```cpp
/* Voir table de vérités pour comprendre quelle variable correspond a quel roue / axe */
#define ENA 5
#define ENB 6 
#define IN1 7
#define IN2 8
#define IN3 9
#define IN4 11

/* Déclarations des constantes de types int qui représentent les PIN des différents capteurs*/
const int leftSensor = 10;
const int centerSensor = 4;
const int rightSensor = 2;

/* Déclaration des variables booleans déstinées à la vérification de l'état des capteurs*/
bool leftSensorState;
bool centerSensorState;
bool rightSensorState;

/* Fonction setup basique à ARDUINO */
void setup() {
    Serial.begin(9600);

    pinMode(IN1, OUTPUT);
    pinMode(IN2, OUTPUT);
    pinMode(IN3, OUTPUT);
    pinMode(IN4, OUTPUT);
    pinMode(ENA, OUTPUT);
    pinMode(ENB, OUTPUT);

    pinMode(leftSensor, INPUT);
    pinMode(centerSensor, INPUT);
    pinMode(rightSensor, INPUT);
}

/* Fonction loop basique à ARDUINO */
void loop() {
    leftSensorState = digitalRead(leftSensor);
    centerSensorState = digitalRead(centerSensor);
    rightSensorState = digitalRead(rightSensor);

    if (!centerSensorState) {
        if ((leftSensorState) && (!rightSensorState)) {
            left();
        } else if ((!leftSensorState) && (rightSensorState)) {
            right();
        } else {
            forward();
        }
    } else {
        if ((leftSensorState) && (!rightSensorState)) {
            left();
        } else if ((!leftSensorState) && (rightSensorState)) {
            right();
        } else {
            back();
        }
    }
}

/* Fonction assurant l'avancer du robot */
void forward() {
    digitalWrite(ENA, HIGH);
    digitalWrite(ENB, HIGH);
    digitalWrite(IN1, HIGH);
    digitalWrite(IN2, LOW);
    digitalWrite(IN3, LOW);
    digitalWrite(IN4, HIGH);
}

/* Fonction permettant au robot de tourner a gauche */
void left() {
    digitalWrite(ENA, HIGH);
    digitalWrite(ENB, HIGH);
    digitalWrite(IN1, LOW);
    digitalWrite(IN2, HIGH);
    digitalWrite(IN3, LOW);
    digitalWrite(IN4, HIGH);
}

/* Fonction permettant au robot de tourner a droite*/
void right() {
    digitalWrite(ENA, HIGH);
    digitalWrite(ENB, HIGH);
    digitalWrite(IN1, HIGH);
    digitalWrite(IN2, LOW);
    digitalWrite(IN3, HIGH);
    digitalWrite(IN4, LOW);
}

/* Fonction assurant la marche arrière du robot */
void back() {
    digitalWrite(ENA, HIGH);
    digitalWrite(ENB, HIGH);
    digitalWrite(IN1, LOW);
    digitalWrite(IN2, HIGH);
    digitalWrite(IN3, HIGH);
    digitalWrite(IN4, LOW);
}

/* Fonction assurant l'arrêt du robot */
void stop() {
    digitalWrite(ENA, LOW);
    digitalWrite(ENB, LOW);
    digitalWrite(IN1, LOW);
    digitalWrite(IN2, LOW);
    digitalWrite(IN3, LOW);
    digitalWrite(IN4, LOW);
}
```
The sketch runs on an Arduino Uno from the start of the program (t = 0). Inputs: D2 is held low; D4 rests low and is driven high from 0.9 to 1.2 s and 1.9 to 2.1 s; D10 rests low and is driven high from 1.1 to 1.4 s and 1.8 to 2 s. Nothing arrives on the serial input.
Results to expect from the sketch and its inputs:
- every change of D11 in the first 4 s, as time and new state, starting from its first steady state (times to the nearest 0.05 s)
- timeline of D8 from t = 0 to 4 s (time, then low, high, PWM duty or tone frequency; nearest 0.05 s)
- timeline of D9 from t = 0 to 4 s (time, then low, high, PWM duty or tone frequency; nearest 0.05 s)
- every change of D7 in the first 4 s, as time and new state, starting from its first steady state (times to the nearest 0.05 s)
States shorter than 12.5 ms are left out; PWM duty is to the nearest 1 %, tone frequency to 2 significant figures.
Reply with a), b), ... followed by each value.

a) 0 s high; 0.9 s low; 1.1 s high; 2 s low; 2.1 s high
b) 0 s low; 0.9 s high; 1.4 s low; 1.8 s high; 2.1 s low
c) 0 s low; 0.9 s high; 1.1 s low; 2 s high; 2.1 s low
d) 0 s high; 0.9 s low; 1.4 s high; 1.8 s low; 2.1 s high
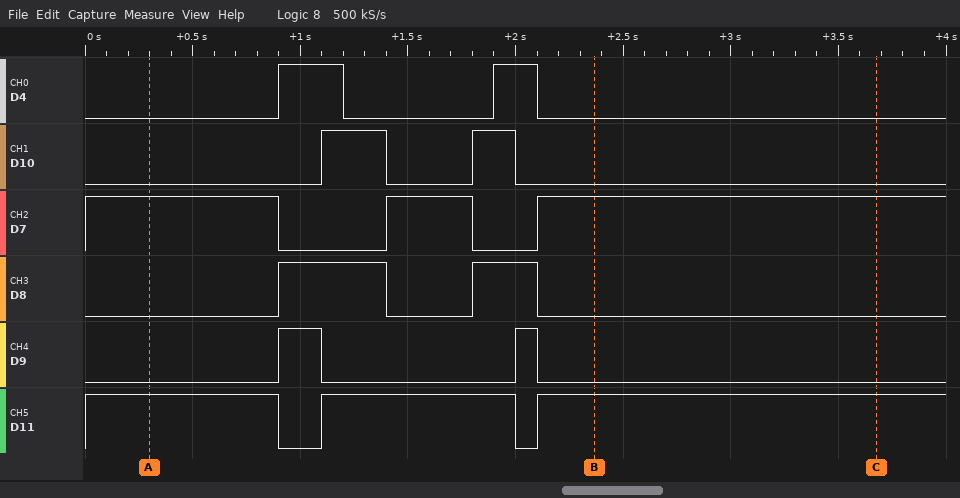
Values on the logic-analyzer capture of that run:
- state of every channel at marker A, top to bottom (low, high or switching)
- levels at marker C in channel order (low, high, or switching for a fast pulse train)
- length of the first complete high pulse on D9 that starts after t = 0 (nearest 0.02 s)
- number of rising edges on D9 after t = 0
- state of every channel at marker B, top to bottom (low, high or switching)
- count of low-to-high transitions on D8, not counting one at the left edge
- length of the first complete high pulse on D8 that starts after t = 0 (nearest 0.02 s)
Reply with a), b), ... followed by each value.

a) D4 low, D10 low, D7 high, D8 low, D9 low, D11 high
b) D4 low, D10 low, D7 high, D8 low, D9 low, D11 high
c) 0.20 s
d) 2
e) D4 low, D10 low, D7 high, D8 low, D9 low, D11 high
f) 2
g) 0.50 s
